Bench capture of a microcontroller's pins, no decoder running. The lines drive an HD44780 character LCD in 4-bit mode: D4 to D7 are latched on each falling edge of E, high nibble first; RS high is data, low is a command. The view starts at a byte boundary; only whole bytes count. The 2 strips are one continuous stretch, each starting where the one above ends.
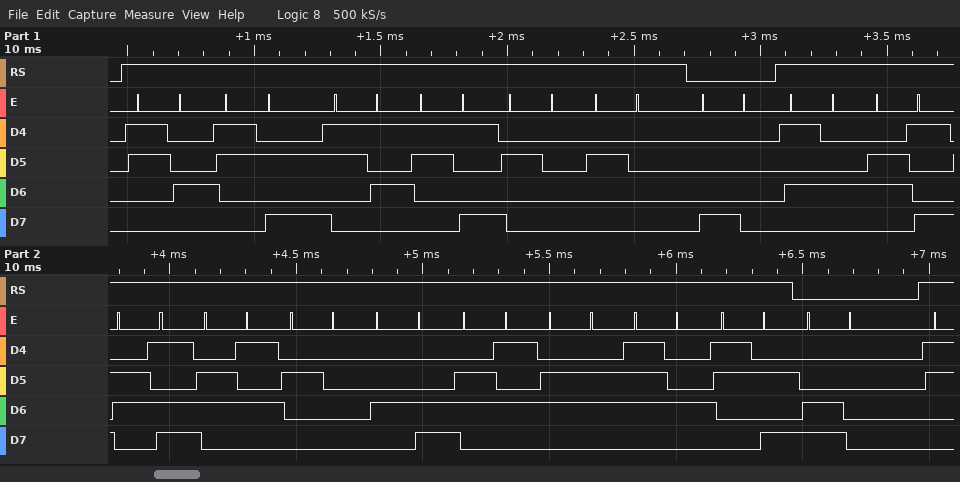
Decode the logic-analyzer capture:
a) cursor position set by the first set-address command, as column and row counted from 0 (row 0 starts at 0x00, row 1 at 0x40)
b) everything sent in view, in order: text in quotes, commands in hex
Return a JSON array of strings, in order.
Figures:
["column 0, row 0", "\"4:59  \" 0x80 \"Time Left:\" 0xC0"]
